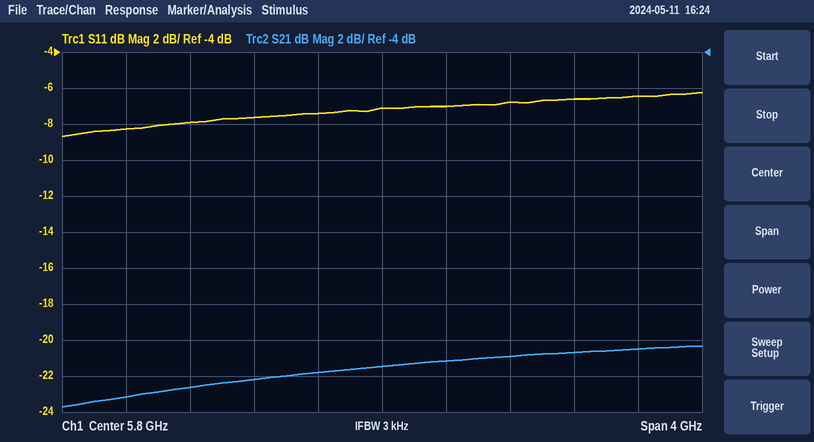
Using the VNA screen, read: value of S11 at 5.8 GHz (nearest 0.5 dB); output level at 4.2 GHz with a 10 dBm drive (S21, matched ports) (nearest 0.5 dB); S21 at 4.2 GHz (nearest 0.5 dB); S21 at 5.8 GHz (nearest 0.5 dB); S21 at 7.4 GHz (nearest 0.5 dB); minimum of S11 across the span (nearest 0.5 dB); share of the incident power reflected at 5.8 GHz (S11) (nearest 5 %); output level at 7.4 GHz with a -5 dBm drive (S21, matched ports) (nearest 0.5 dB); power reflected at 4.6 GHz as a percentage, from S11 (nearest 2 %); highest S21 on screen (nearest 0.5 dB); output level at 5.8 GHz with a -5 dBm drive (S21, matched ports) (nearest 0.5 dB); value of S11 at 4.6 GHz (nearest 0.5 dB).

-7.0 dB
-13.0 dBm
-23.0 dB
-21.5 dB
-20.5 dB
-8.5 dB
20 %
-25.5 dBm
16 %
-20.5 dB
-26.5 dBm
-8.0 dB
